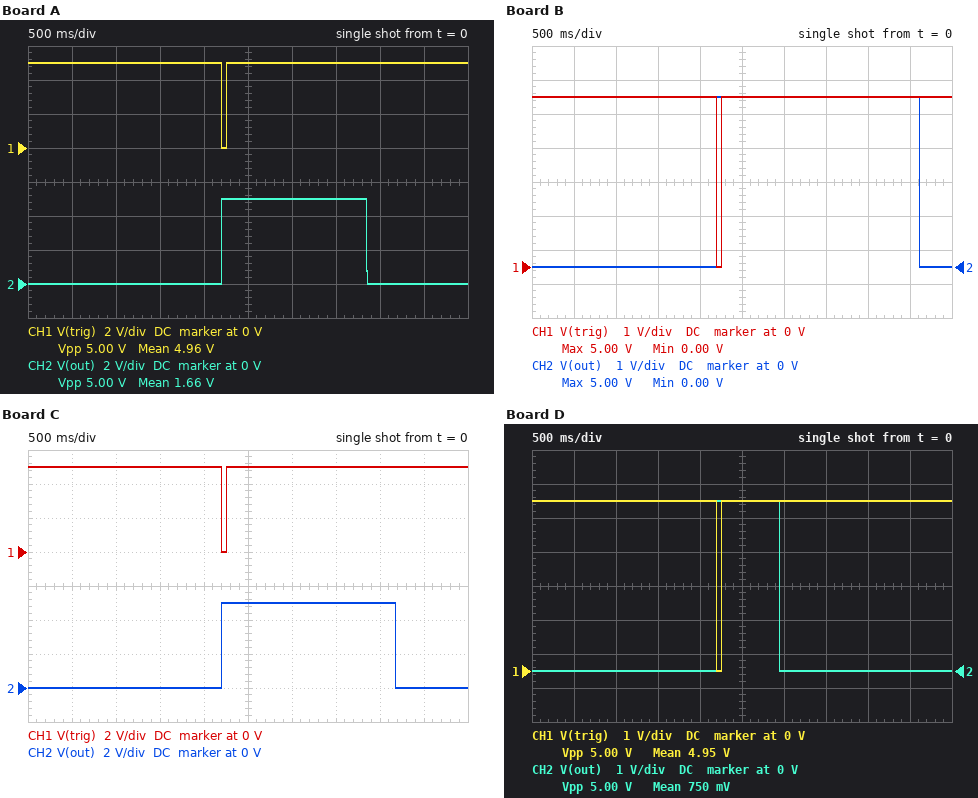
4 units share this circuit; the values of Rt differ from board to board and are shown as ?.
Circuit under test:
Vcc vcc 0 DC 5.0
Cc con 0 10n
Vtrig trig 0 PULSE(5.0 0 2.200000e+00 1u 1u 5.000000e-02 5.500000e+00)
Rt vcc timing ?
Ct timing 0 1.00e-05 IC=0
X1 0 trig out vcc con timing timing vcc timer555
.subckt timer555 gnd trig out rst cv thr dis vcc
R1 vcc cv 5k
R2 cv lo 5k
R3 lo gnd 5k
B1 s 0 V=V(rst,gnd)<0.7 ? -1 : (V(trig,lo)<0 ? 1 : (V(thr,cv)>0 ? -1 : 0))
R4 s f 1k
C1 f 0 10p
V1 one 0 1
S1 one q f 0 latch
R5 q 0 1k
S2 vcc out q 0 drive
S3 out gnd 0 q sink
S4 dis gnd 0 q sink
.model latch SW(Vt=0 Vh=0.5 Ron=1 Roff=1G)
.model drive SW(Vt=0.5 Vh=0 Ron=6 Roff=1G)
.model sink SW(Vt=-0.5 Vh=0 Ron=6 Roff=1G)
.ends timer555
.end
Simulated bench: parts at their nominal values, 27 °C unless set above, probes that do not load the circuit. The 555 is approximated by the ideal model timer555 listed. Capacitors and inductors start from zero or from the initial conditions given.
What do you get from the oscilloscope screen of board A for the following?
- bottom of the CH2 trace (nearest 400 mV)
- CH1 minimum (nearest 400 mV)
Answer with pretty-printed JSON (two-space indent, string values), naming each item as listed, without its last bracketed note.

{
  "bottom of the CH2 trace": "0 V",
  "CH1 minimum": "0 V"
}
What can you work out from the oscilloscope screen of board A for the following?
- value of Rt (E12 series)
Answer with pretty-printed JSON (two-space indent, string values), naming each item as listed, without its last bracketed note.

{
  "value of Rt": "150 kΩ"
}
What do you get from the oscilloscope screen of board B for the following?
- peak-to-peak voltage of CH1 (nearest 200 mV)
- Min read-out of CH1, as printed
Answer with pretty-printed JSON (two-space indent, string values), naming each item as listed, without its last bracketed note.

{
  "peak-to-peak voltage of CH1": "5.0 V",
  "Min read-out of CH1, as printed": "0.00 V"
}
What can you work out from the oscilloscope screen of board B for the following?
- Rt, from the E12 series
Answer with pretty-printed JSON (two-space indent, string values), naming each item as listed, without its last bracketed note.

{
  "Rt, from the E12 series": "220 kΩ"
}
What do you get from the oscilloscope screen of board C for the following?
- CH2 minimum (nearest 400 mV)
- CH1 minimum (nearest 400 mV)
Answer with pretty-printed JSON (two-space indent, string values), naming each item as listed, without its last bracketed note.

{
  "CH2 minimum": "0 V",
  "CH1 minimum": "0 V"
}
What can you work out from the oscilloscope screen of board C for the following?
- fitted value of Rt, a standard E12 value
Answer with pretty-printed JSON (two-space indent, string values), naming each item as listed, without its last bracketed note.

{
  "fitted value of Rt, a standard E12 value": "180 kΩ"
}
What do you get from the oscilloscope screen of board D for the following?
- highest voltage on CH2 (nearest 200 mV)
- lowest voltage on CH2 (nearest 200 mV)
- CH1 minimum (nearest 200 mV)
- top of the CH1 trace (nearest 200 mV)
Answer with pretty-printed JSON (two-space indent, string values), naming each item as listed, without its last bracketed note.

{
  "highest voltage on CH2": "5.0 V",
  "lowest voltage on CH2": "0 V",
  "CH1 minimum": "0 V",
  "top of the CH1 trace": "5.0 V"
}
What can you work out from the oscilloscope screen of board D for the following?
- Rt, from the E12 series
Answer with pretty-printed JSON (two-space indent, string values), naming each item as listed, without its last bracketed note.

{
  "Rt, from the E12 series": "68 kΩ"
}
